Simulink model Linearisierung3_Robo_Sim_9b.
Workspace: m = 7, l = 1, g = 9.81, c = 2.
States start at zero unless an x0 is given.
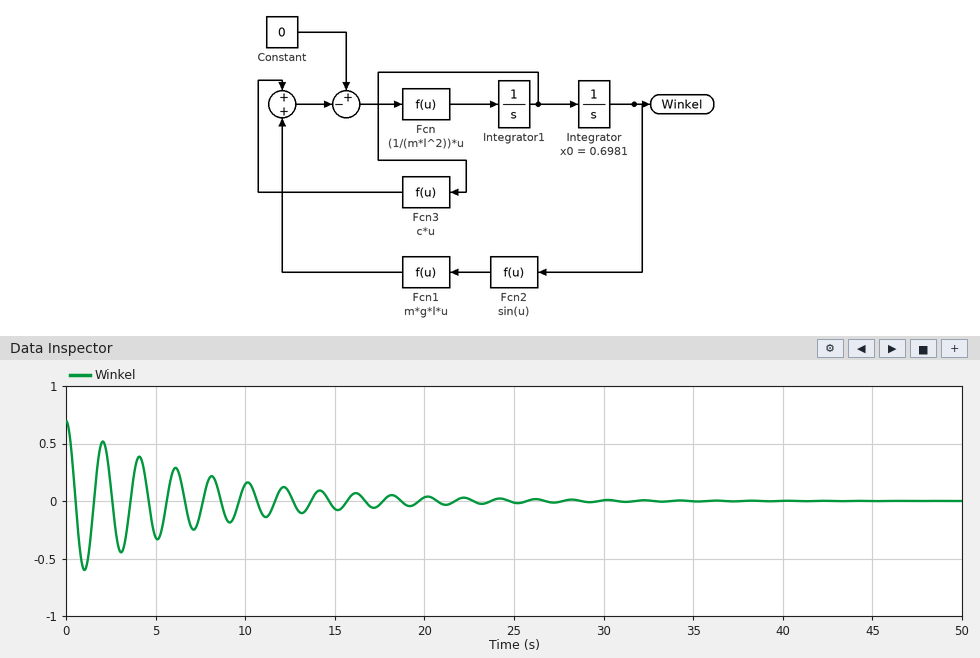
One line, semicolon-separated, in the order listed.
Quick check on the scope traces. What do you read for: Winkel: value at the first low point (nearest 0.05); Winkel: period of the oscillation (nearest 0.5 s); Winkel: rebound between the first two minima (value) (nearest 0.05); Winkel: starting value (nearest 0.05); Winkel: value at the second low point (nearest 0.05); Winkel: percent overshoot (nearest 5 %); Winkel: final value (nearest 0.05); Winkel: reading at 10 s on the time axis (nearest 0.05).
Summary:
-0.60; 2.0 s; 0.50; 0.70; -0.45; 85 %; 0.00; 0.15
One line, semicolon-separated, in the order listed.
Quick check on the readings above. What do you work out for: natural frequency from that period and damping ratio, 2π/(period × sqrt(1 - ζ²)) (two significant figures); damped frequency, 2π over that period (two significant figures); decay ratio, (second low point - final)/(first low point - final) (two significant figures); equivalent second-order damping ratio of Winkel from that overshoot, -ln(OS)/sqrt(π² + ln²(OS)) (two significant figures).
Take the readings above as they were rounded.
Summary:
3.1 rad/s; 3.1 rad/s; 0.75; 0.052
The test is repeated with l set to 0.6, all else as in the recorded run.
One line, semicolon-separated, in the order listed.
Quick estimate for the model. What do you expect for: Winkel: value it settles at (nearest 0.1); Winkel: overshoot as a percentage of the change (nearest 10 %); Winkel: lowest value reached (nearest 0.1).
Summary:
0.0; 70 %; -0.5
